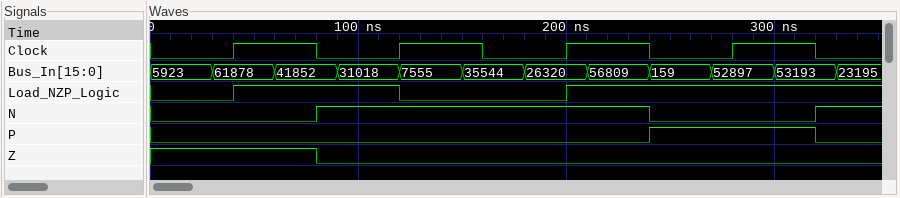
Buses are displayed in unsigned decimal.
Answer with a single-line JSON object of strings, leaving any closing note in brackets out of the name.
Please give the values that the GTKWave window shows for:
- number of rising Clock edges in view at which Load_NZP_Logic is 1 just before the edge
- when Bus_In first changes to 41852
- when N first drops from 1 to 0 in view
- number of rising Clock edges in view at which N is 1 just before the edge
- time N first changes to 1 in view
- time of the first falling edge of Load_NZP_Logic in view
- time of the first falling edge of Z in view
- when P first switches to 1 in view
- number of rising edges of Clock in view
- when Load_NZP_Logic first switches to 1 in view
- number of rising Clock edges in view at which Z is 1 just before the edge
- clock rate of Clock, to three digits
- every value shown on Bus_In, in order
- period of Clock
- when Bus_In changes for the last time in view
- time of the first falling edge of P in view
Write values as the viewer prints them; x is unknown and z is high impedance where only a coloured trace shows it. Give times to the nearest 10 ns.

{"number of rising Clock edges in view at which Load_NZP_Logic is 1 just before the edge": "2", "when Bus_In first changes to 41852": "60 ns", "when N first drops from 1 to 0 in view": "240 ns", "number of rising Clock edges in view at which N is 1 just before the edge": "2", "time N first changes to 1 in view": "80 ns", "time of the first falling edge of Load_NZP_Logic in view": "120 ns", "time of the first falling edge of Z in view": "80 ns", "when P first switches to 1 in view": "240 ns", "number of rising edges of Clock in view": "4", "when Load_NZP_Logic first switches to 1 in view": "40 ns", "number of rising Clock edges in view at which Z is 1 just before the edge": "1", "clock rate of Clock, to three digits": "12.5 MHz", "every value shown on Bus_In, in order": "5923, 61878, 41852, 31018, 7555, 35544, 26320, 56809, 159, 52897, 53193, 23195", "period of Clock": "80 ns", "when Bus_In changes for the last time in view": "330 ns", "time of the first falling edge of P in view": "320 ns"}
